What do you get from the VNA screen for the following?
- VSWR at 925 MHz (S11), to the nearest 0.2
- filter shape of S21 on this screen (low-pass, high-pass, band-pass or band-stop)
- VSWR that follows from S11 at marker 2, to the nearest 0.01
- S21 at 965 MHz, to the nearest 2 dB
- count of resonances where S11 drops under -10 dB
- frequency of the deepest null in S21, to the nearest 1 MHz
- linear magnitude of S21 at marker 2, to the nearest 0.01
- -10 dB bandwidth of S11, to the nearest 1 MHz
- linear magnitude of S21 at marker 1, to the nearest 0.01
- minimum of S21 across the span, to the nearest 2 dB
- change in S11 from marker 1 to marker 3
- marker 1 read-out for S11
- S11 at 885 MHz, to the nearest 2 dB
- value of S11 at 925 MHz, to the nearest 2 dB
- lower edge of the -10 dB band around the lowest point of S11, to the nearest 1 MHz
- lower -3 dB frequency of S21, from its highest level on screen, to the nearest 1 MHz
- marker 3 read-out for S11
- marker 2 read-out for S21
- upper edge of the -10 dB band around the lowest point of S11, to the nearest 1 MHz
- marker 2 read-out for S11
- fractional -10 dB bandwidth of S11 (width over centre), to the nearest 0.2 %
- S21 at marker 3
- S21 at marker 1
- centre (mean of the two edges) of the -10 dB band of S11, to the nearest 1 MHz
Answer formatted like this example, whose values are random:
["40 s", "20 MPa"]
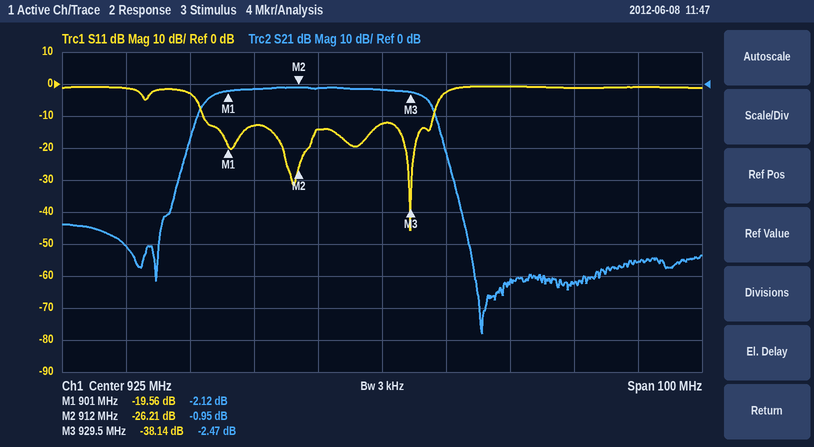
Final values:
["1.6", "band-pass", "1.10", "-56 dB", "4", "941 MHz", "0.90", "36 MHz", "0.78", "-78 dB", "-18.58 dB", "-19.56 dB", "-2 dB", "-12 dB", "897 MHz", "898 MHz", "-38.14 dB", "-0.95 dB", "933 MHz", "-26.21 dB", "4.0 %", "-2.47 dB", "-2.12 dB", "915 MHz"]
